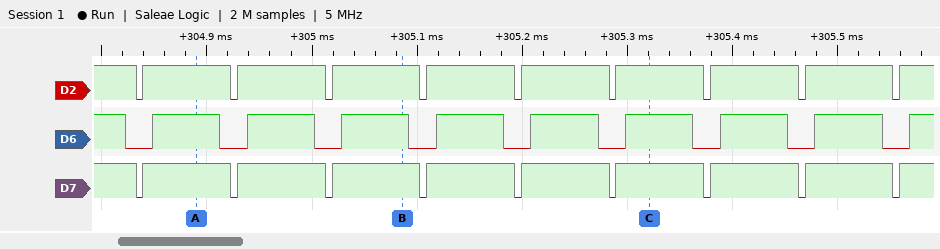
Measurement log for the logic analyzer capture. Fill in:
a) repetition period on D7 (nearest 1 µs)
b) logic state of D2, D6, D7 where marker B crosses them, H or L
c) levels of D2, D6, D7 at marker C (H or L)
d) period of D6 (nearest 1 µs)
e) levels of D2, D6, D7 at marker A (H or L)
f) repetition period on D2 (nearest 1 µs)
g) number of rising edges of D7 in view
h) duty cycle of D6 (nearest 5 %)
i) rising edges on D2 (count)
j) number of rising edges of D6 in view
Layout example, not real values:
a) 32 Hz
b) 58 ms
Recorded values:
a) 90 µs
b) D2=H, D6=H, D7=H
c) D2=H, D6=H, D7=H
d) 90 µs
e) D2=H, D6=H, D7=H
f) 90 µs
g) 9
h) 70 %
i) 9
j) 9
